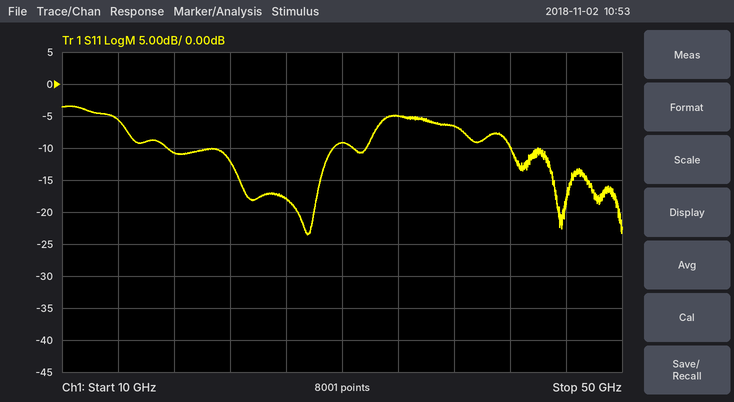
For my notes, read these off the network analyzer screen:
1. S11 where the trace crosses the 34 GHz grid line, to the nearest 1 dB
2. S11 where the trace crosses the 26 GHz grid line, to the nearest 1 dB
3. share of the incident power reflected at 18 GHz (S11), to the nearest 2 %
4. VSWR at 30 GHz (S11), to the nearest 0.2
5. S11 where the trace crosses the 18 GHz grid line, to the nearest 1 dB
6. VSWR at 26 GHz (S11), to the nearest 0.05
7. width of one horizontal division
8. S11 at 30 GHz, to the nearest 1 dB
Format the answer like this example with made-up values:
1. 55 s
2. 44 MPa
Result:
1. -5 dB
2. -18 dB
3. 8 %
4. 2.0
5. -11 dB
6. 1.30
7. 4 GHz
8. -9 dB
